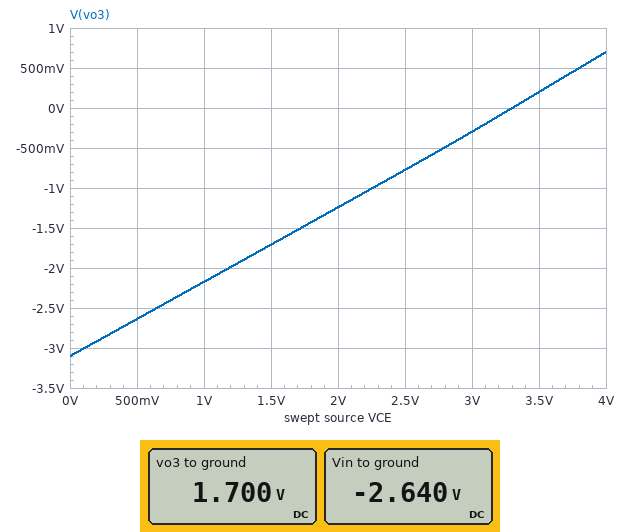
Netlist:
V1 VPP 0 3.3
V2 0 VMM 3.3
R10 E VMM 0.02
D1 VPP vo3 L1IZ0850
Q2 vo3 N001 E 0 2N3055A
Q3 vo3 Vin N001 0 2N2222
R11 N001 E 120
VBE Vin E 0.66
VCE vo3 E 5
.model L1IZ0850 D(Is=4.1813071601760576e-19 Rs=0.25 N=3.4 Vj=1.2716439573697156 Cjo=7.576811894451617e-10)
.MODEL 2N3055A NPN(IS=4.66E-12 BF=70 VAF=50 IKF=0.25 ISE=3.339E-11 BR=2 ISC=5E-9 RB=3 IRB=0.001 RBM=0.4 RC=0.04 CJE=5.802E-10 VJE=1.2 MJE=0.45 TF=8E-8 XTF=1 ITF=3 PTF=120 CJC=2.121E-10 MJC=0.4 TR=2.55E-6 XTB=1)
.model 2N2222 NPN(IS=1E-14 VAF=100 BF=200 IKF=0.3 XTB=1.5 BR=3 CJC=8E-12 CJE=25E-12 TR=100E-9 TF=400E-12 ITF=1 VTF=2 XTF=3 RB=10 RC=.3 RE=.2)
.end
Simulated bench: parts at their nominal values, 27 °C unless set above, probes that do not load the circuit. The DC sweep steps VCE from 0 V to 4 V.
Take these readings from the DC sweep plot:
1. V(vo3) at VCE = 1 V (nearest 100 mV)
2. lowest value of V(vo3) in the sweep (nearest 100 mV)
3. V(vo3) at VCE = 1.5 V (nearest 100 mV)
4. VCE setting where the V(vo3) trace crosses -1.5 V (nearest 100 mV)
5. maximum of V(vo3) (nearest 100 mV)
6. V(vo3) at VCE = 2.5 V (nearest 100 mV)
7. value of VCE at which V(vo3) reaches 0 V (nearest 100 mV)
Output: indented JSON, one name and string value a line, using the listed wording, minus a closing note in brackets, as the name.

{
  "V(vo3) at VCE = 1 V": "-2.2 V",
  "lowest value of V(vo3) in the sweep": "-3.1 V",
  "V(vo3) at VCE = 1.5 V": "-1.7 V",
  "VCE setting where the V(vo3) trace crosses -1.5 V": "1.7 V",
  "maximum of V(vo3)": "700 mV",
  "V(vo3) at VCE = 2.5 V": "-800 mV",
  "value of VCE at which V(vo3) reaches 0 V": "3.3 V"
}
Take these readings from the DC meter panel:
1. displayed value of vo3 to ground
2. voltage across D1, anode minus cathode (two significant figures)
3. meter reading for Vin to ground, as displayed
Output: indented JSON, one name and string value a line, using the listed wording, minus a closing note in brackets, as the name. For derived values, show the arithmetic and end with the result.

{
  "displayed value of vo3 to ground": "1.700 V",
  "voltage across D1, anode minus cathode": "3.3 V - 1.7 V = 1.6 V",
  "meter reading for Vin to ground, as displayed": "-2.640 V"
}
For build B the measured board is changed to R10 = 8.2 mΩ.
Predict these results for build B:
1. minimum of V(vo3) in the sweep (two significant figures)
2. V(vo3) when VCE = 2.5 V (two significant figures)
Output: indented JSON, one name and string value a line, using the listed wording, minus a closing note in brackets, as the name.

{
  "minimum of V(vo3) in the sweep": "-3.2 V",
  "V(vo3) when VCE = 2.5 V": "-790 mV"
}
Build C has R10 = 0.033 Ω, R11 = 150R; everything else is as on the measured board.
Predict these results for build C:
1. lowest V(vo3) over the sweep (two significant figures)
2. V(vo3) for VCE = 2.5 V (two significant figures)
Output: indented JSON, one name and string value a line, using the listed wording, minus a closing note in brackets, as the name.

{
  "lowest V(vo3) over the sweep": "-3.0 V",
  "V(vo3) for VCE = 2.5 V": "-760 mV"
}
